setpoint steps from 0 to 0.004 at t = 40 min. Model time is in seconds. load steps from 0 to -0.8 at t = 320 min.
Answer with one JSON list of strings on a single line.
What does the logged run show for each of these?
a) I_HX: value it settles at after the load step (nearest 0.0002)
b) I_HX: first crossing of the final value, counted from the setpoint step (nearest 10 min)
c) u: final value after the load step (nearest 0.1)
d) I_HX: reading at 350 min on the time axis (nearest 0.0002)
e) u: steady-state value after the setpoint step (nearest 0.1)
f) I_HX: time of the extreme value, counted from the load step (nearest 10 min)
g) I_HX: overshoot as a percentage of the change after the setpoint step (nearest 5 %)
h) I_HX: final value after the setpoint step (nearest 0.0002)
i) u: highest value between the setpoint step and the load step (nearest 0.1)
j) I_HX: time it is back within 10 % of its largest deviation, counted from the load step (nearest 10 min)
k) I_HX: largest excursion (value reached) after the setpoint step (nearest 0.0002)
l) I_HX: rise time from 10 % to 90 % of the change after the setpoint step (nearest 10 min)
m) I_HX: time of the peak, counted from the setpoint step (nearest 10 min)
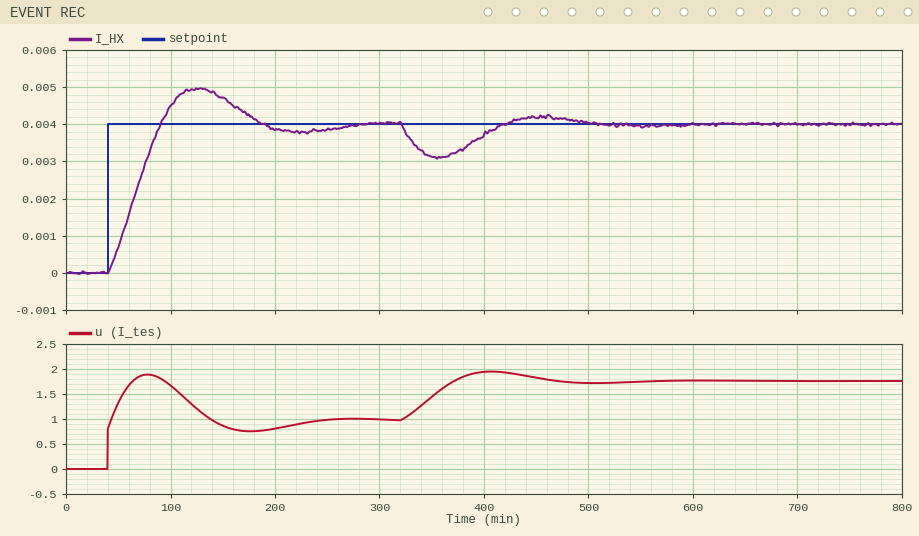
["0.0040", "50 min", "1.8", "0.0032", "1.0", "40 min", "25 %", "0.0040", "1.9", "170 min", "0.0050", "40 min", "90 min"]
